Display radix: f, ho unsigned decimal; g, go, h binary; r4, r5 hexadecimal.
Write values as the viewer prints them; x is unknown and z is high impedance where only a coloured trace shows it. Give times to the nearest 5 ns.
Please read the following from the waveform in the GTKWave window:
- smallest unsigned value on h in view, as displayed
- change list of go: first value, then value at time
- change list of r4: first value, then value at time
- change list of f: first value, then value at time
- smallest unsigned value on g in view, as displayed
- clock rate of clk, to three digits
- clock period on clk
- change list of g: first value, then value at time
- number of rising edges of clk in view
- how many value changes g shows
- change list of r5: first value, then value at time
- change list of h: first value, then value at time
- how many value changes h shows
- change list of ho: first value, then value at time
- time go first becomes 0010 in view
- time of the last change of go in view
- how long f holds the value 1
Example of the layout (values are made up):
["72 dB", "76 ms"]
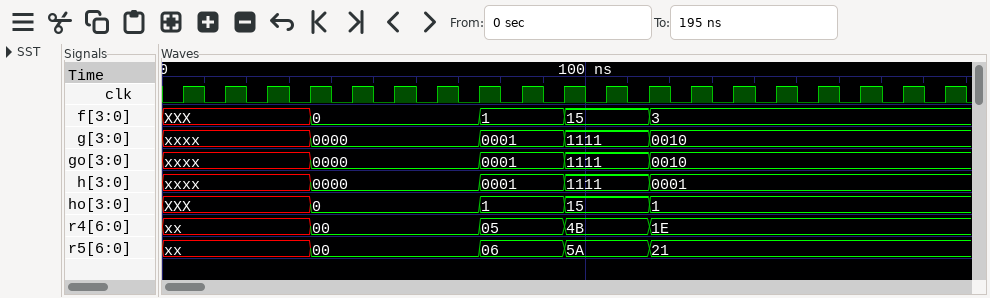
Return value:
["0000", "xxxx, 0000 at 35 ns, 0001 at 75 ns, 1111 at 95 ns, 0010 at 115 ns", "xx, 00 at 35 ns, 05 at 75 ns, 4B at 95 ns, 1E at 115 ns", "XXX, 0 at 35 ns, 1 at 75 ns, 15 at 95 ns, 3 at 115 ns", "0000", "100 MHz", "10 ns", "xxxx, 0000 at 35 ns, 0001 at 75 ns, 1111 at 95 ns, 0010 at 115 ns", "19", "4", "xx, 00 at 35 ns, 06 at 75 ns, 5A at 95 ns, 21 at 115 ns", "xxxx, 0000 at 35 ns, 0001 at 75 ns, 1111 at 95 ns, 0001 at 115 ns", "4", "XXX, 0 at 35 ns, 1 at 75 ns, 15 at 95 ns, 1 at 115 ns", "115 ns", "115 ns", "20 ns"]
